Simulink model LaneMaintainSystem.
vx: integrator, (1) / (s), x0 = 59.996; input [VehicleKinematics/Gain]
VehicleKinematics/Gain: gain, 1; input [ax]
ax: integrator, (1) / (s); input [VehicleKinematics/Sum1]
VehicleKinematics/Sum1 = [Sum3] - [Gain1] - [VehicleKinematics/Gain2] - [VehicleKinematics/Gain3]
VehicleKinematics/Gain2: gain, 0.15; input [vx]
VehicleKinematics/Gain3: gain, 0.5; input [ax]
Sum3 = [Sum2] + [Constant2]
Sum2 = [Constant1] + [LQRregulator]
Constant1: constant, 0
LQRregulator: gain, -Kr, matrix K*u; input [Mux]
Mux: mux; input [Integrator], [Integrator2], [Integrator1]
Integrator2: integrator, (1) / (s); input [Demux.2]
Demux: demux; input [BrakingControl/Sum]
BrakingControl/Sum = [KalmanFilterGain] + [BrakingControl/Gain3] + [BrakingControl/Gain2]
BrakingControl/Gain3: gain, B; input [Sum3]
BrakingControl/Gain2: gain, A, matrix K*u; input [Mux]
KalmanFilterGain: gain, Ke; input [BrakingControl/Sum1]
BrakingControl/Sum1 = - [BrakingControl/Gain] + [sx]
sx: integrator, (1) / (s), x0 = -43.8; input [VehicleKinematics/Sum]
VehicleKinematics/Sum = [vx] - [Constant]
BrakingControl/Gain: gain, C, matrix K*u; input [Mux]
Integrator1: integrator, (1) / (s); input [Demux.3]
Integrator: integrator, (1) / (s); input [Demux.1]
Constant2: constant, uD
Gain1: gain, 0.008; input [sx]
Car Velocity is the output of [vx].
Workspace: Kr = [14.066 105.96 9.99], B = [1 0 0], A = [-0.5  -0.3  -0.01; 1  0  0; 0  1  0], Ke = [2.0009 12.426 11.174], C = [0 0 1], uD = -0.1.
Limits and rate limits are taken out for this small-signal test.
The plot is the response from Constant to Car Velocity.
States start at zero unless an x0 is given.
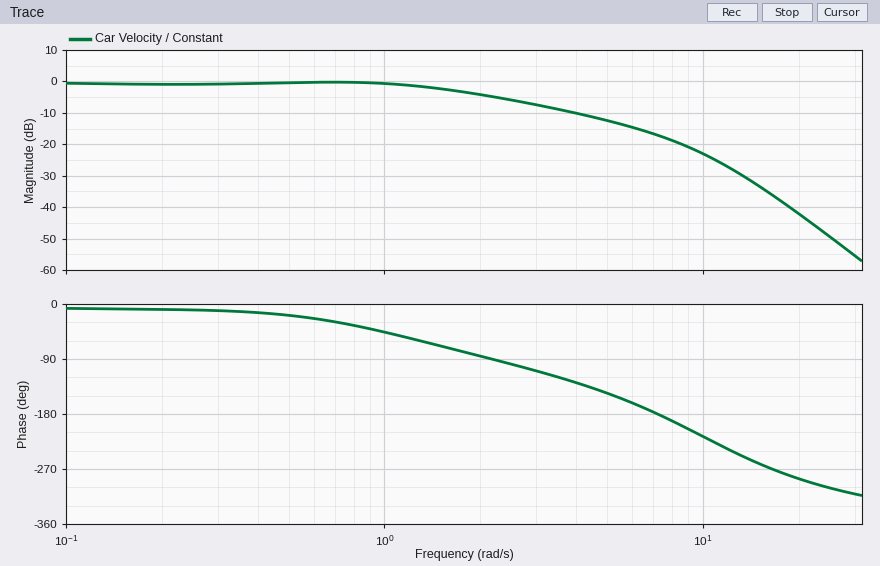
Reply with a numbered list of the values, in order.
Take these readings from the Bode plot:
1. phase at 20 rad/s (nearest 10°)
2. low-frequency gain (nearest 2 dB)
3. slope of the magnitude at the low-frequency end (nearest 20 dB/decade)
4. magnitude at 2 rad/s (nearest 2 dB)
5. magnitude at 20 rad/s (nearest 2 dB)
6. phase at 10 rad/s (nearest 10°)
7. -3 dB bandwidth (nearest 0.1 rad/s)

1. -290°
2. 0 dB
3. 0 dB/decade
4. -4 dB
5. -42 dB
6. -220°
7. 1.9 rad/s
